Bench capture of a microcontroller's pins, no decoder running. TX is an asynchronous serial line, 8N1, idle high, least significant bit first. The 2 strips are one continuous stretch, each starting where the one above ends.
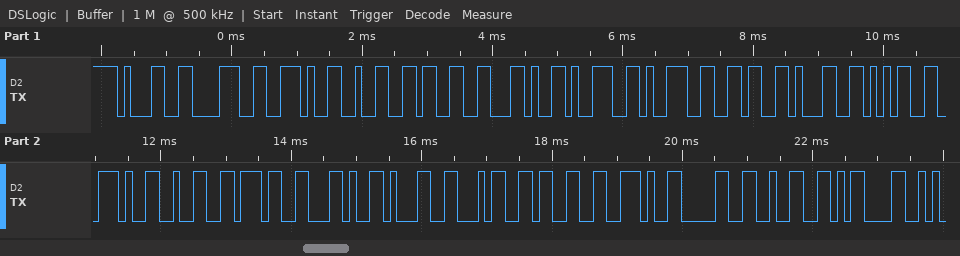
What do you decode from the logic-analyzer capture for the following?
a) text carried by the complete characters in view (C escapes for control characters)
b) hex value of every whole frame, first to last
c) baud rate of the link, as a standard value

"18.23,99615.27,143.02\r"
31 38 2E 32 33 2C 39 39 36 31 35 2E 32 37 2C 31 34 33 2E 30 32 0D
9600 baud
